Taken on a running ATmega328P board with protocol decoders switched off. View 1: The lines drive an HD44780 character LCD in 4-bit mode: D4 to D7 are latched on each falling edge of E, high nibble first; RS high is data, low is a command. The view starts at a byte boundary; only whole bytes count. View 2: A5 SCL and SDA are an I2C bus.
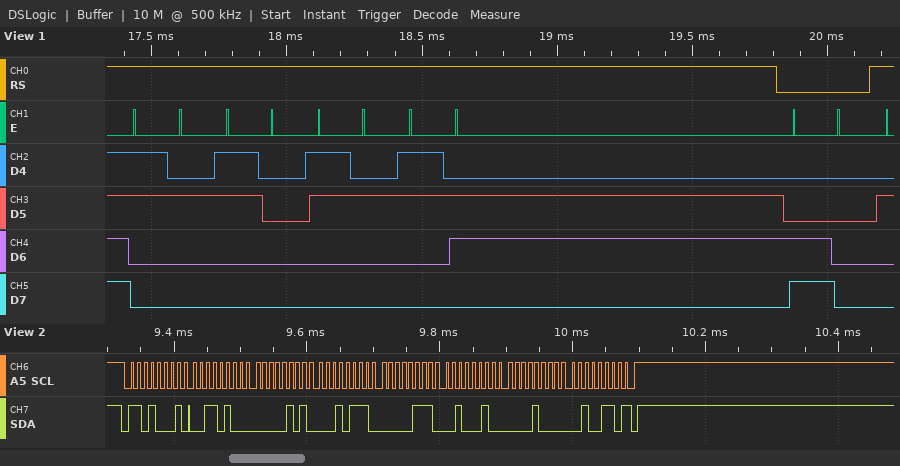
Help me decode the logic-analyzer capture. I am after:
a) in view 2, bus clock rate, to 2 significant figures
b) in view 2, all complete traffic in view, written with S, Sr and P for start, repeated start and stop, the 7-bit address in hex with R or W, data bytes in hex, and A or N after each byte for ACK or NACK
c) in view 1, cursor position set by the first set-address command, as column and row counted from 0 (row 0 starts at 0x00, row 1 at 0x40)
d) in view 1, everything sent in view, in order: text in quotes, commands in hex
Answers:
100 kHz
S 68R A 34 A 05 A 17 A 07 A 22 A 08 A 26 N P
column 0, row 1
"2026" 0xC0
